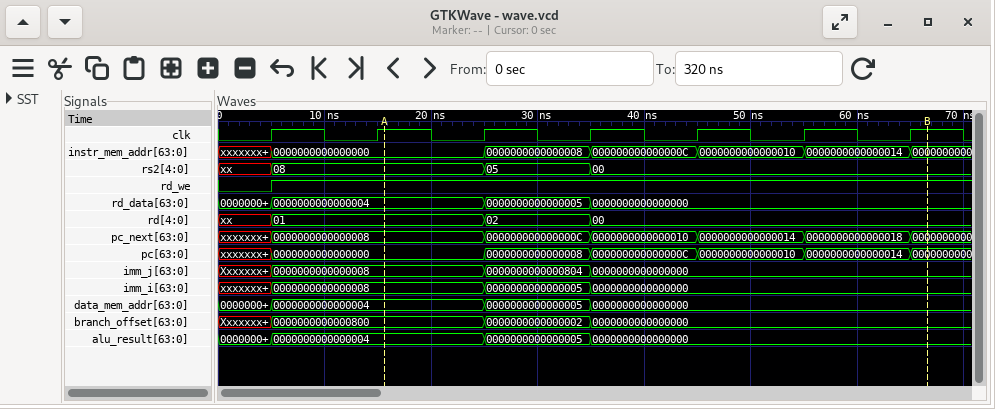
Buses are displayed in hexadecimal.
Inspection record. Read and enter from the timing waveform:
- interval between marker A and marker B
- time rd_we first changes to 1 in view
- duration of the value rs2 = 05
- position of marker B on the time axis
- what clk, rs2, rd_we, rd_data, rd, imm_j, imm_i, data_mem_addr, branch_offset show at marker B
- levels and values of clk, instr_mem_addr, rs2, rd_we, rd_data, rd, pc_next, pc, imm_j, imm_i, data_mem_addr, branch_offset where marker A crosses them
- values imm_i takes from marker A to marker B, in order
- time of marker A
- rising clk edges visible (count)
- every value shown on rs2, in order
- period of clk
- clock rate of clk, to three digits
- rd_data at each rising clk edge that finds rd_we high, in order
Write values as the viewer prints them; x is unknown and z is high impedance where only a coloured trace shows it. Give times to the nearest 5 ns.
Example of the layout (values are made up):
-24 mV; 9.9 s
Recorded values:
50 ns; 5 ns; 10 ns; 65 ns; clk=1, rs2=00, rd_we=1, rd_data=0000000000000000, rd=00, imm_j=0000000000000000, imm_i=0000000000000000, data_mem_addr=0000000000000000, branch_offset=0000000000000000; clk=1, instr_mem_addr=0000000000000000, rs2=08, rd_we=1, rd_data=0000000000000004, rd=01, pc_next=0000000000000008, pc=0000000000000000, imm_j=0000000000000008, imm_i=0000000000000008, data_mem_addr=0000000000000004, branch_offset=0000000000000800; 0000000000000008, 0000000000000005, 0000000000000000; 15 ns; 7; xx, 08, 05, 00; 10 ns; 100 MHz; 0000000000000004, 0000000000000004, 0000000000000005, 0000000000000000, 0000000000000000, 0000000000000000
